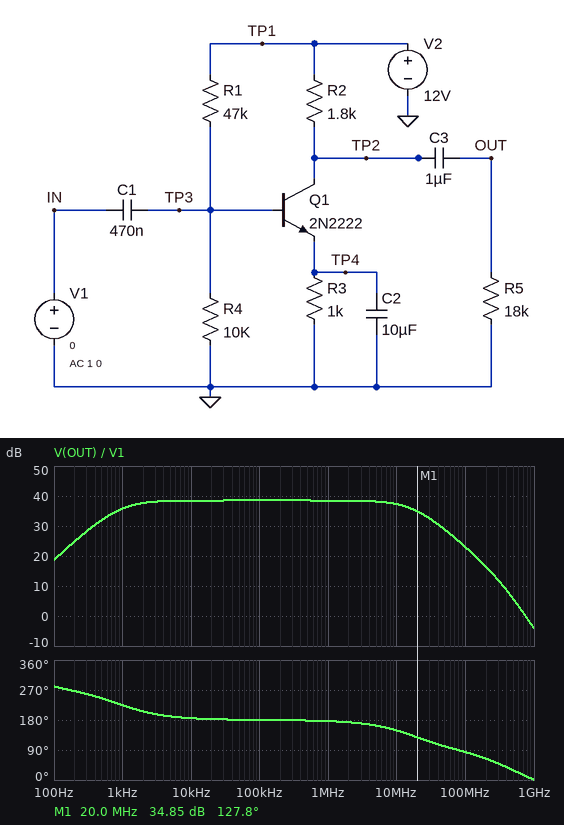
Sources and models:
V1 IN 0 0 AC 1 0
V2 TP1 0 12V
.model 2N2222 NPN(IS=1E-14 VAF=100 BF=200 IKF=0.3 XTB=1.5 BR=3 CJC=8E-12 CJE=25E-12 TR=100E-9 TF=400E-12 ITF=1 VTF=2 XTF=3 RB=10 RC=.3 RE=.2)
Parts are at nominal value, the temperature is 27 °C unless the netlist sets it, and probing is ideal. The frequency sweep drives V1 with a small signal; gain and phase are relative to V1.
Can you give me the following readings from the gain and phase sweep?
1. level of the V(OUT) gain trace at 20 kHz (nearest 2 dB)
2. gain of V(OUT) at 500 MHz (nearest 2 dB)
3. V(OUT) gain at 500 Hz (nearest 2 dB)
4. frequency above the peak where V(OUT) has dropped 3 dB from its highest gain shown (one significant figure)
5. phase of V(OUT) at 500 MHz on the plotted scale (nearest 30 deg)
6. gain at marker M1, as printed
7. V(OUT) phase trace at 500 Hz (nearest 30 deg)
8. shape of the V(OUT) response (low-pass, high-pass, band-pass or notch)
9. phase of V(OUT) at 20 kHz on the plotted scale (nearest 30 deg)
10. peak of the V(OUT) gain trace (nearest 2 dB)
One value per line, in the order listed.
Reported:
38 dB
6 dB
32 dB
20 MHz
30 deg
34.85 dB
240 deg
band-pass
180 deg
38 dB
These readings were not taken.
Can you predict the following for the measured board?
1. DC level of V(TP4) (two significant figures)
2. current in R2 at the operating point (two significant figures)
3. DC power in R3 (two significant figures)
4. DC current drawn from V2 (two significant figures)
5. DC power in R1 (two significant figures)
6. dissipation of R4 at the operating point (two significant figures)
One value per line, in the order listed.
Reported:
1.4 V
1.4 mA
1.9 mW
1.6 mA
2.1 mW
420 µW
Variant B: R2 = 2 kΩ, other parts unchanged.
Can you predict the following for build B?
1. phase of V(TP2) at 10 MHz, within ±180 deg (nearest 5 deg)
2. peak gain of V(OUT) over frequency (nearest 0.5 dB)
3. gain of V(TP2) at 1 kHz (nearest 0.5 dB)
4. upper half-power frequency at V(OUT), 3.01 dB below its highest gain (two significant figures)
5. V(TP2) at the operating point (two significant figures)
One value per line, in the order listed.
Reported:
145 deg
39.5 dB
36.5 dB
16 MHz
9.2 V
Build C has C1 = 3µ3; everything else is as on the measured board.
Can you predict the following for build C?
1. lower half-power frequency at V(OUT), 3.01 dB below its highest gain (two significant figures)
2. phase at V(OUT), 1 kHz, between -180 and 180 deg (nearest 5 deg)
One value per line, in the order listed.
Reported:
850 Hz
-140 deg
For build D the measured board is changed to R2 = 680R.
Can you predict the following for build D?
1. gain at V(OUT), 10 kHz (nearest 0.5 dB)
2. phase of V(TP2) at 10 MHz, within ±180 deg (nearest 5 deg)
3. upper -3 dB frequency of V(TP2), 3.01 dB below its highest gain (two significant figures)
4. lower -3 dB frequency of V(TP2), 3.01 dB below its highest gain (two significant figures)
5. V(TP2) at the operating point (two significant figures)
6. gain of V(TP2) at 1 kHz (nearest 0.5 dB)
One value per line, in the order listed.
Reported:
30.5 dB
165 deg
43 MHz
940 Hz
11 V
28.0 dB
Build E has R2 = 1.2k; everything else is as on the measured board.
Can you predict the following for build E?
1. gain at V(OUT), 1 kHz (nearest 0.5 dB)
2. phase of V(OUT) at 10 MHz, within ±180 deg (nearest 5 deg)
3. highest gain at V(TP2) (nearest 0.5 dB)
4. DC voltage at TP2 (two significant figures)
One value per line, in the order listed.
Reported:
32.5 dB
155 deg
35.5 dB
10 V
